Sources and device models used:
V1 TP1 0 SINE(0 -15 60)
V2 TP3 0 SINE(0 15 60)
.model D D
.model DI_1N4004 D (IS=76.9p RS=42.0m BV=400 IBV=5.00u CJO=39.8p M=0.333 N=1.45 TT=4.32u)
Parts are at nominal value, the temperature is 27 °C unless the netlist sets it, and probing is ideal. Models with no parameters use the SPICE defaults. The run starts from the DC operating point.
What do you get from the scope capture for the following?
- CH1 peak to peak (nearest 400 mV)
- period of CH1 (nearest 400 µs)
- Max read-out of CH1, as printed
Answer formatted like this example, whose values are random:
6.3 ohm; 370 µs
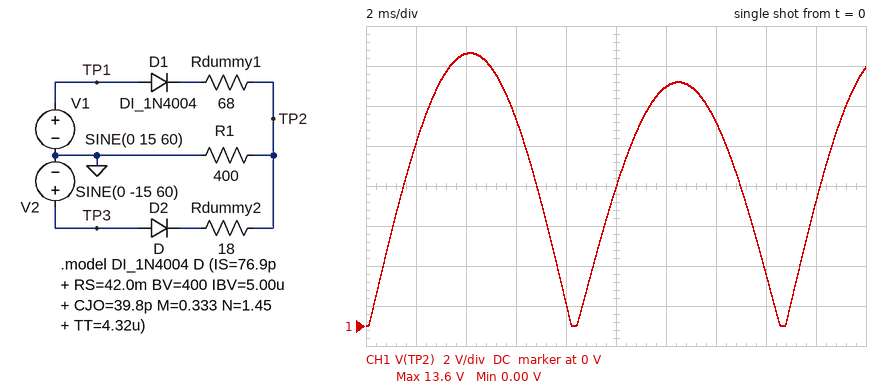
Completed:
13.6 V; 8.4 ms; 13.6 V
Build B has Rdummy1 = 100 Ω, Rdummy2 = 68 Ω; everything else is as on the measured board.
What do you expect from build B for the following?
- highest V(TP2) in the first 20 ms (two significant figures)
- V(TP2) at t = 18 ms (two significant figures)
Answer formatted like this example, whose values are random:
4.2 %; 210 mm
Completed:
12 V; 5.6 V
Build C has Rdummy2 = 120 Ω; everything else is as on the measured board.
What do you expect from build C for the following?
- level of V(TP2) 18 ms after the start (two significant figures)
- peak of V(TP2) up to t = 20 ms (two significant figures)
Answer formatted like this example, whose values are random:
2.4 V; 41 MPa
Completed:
5.0 V; 12 V
